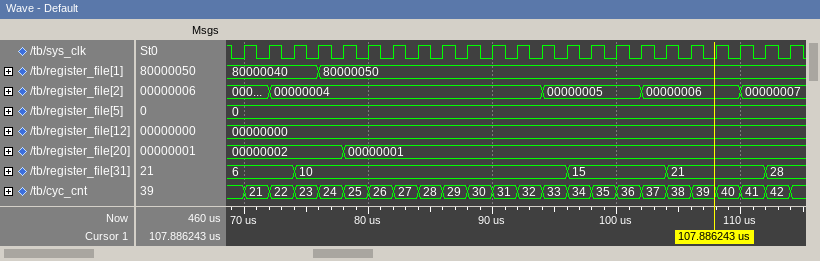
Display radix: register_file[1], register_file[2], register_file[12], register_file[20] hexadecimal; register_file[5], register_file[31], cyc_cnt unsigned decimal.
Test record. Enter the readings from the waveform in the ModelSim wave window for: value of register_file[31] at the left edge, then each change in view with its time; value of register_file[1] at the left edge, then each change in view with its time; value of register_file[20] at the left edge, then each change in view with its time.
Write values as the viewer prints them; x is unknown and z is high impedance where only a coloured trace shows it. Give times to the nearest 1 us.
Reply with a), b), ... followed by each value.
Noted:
a) 6, 10 at 74 us, 15 at 96 us, 21 at 104 us, 28 at 112 us
b) 80000040, 80000050 at 76 us
c) 00000002, 00000001 at 78 us
